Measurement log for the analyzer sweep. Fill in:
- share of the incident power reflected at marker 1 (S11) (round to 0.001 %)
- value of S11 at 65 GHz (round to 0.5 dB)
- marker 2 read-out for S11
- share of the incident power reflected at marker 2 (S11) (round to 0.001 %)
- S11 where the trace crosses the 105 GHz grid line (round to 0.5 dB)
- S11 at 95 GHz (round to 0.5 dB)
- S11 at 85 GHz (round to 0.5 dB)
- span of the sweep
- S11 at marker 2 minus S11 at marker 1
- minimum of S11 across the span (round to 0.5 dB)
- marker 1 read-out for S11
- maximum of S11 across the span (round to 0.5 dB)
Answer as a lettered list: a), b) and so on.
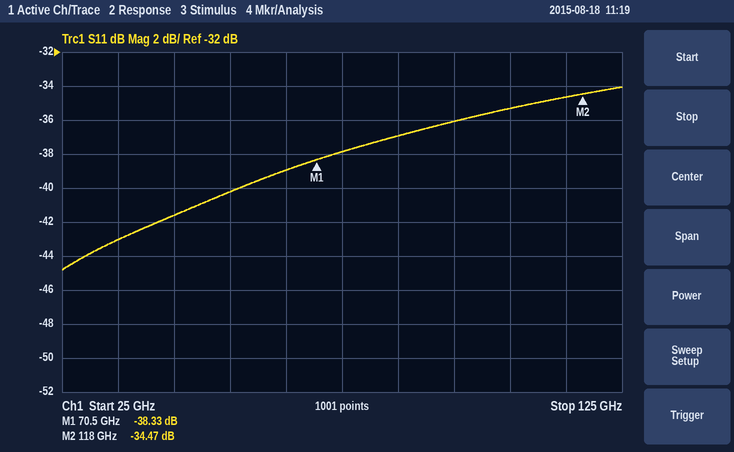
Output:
a) 0.015 %
b) -39.0 dB
c) -34.47 dB
d) 0.036 %
e) -35.5 dB
f) -36.0 dB
g) -37.0 dB
h) 100 GHz
i) 3.86 dB
j) -45.0 dB
k) -38.33 dB
l) -34.0 dB
